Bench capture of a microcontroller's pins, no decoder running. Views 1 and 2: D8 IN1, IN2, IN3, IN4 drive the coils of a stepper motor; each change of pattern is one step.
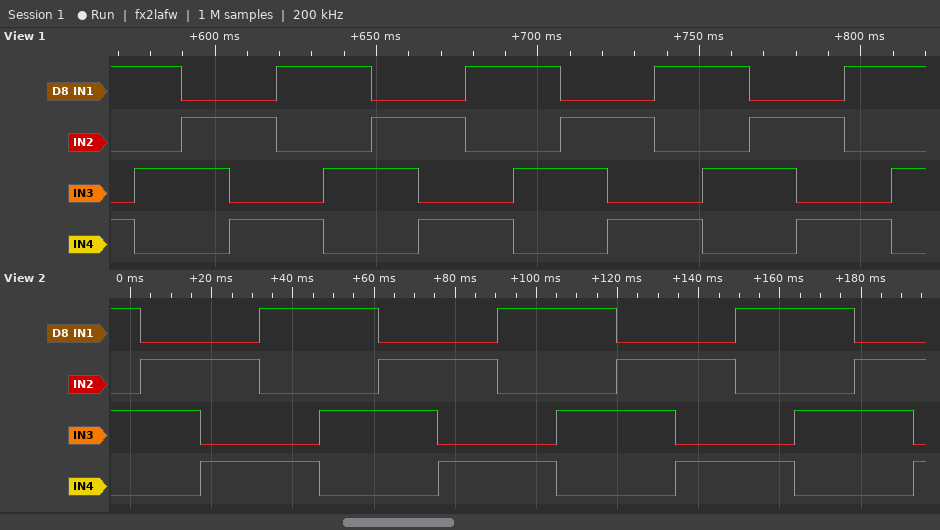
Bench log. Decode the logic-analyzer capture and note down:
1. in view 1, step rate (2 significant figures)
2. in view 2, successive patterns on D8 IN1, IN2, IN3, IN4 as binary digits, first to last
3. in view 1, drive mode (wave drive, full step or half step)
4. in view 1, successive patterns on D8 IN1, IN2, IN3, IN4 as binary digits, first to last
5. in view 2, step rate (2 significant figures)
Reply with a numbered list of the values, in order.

1. 68 steps/s
2. 1010 0110 0101 1001 1010 0110 0101 1001 1010 0110 0101 1001 1010 0110 0101
3. full step
4. 1001 1010 0110 0101 1001 1010 0110 0101 1001 1010 0110 0101 1001 1010 0110 0101 1001 1010
5. 68 steps/s
